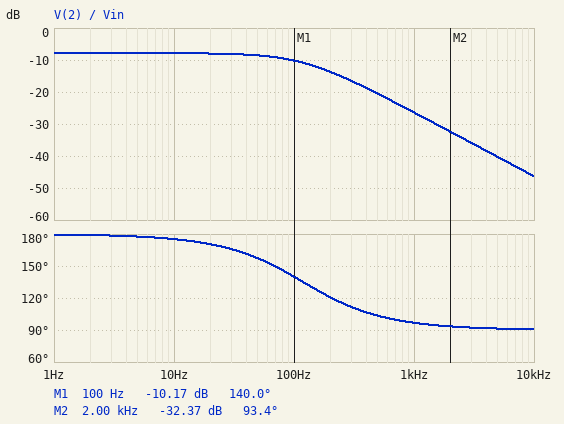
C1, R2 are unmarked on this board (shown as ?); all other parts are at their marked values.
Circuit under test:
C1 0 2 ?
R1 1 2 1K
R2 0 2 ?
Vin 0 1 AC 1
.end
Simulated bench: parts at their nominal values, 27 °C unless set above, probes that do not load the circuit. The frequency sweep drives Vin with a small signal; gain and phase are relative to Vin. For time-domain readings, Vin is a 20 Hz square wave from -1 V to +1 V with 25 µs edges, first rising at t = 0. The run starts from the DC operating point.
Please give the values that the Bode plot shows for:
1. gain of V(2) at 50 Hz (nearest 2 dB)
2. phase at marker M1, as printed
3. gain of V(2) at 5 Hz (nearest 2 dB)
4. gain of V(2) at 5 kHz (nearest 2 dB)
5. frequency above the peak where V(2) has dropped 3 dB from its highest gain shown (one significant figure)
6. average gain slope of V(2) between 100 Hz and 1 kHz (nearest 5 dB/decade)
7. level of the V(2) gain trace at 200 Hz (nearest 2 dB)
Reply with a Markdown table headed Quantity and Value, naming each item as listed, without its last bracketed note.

| Quantity | Value |
|---|---|
| gain of V(2) at 50 Hz | -8 dB |
| phase at marker M1, as printed | 140.0 deg |
| gain of V(2) at 5 Hz | -8 dB |
| gain of V(2) at 5 kHz | -40 dB |
| frequency above the peak where V(2) has dropped 3 dB from its highest gain shown | 100 Hz |
| average gain slope of V(2) between 100 Hz and 1 kHz | -15 dB/decade |
| level of the V(2) gain trace at 200 Hz | -14 dB |
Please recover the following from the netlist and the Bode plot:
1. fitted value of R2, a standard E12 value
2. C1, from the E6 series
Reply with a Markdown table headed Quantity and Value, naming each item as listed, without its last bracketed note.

| Quantity | Value |
|---|---|
| fitted value of R2, a standard E12 value | 680 Ω |
| C1, from the E6 series | 3.3 µF |
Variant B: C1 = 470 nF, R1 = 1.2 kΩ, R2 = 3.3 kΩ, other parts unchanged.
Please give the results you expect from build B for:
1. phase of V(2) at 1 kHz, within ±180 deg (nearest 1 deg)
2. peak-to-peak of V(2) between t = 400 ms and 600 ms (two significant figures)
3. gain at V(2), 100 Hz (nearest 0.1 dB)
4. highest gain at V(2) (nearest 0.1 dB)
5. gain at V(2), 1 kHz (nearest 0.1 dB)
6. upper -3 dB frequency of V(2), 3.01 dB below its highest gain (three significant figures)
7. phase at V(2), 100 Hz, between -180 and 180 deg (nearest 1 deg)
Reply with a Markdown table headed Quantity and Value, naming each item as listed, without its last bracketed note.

| Quantity | Value |
|---|---|
| phase of V(2) at 1 kHz, within ±180 deg | 111 deg |
| peak-to-peak of V(2) between t = 400 ms and 600 ms | 1.5 V |
| gain at V(2), 100 Hz | -3.0 dB |
| highest gain at V(2) | -2.7 dB |
| gain at V(2), 1 kHz | -11.6 dB |
| upper -3 dB frequency of V(2), 3.01 dB below its highest gain | 385 Hz |
| phase at V(2), 100 Hz, between -180 and 180 deg | 165 deg |
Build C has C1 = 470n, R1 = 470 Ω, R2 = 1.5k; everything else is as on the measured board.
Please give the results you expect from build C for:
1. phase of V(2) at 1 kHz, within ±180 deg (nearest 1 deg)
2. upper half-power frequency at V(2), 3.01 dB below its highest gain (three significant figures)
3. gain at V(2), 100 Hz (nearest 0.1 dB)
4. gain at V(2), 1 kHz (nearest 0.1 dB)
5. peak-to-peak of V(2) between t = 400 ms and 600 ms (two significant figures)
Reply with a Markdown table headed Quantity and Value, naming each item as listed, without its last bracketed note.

| Quantity | Value |
|---|---|
| phase of V(2) at 1 kHz, within ±180 deg | 133 deg |
| upper half-power frequency at V(2), 3.01 dB below its highest gain | 946 Hz |
| gain at V(2), 100 Hz | -2.4 dB |
| gain at V(2), 1 kHz | -5.6 dB |
| peak-to-peak of V(2) between t = 400 ms and 600 ms | 1.5 V |
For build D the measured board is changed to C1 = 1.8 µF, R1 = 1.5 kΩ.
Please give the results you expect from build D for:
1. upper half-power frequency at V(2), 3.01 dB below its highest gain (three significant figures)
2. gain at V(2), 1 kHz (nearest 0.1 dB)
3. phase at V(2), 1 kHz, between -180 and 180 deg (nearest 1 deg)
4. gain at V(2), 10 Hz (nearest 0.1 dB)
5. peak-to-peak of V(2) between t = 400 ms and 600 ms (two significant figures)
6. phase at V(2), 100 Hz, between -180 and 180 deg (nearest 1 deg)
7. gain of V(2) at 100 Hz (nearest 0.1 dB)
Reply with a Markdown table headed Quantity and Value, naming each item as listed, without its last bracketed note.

| Quantity | Value |
|---|---|
| upper half-power frequency at V(2), 3.01 dB below its highest gain | 189 Hz |
| gain at V(2), 1 kHz | -24.7 dB |
| phase at V(2), 1 kHz, between -180 and 180 deg | 101 deg |
| gain at V(2), 10 Hz | -10.1 dB |
| peak-to-peak of V(2) between t = 400 ms and 600 ms | 620 mV |
| phase at V(2), 100 Hz, between -180 and 180 deg | 152 deg |
| gain of V(2) at 100 Hz | -11.2 dB |
